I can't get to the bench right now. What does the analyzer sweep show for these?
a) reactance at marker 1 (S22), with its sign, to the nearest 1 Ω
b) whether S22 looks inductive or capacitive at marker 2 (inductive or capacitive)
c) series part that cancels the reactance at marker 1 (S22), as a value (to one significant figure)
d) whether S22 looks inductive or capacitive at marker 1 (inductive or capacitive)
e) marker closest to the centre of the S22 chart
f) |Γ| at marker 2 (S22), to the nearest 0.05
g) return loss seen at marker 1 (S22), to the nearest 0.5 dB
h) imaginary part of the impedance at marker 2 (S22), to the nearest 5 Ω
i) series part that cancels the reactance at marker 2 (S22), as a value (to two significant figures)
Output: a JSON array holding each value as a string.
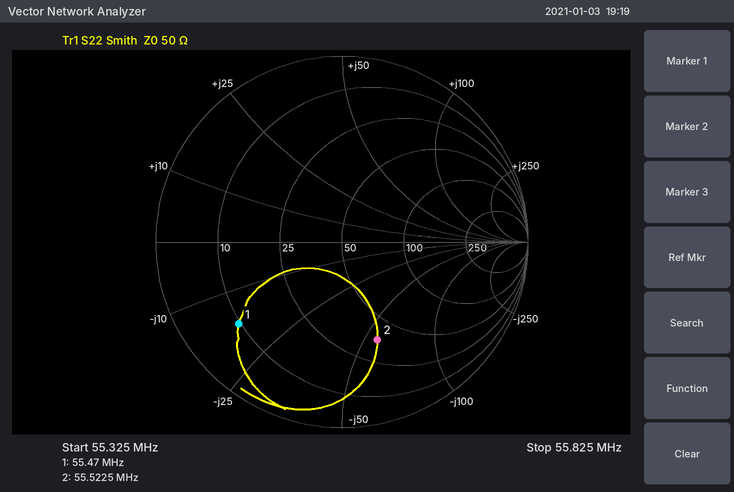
["-17 Ω", "capacitive", "50 nH", "capacitive", "marker 2", "0.55", "3.0 dB", "-55 Ω", "160 nH"]
